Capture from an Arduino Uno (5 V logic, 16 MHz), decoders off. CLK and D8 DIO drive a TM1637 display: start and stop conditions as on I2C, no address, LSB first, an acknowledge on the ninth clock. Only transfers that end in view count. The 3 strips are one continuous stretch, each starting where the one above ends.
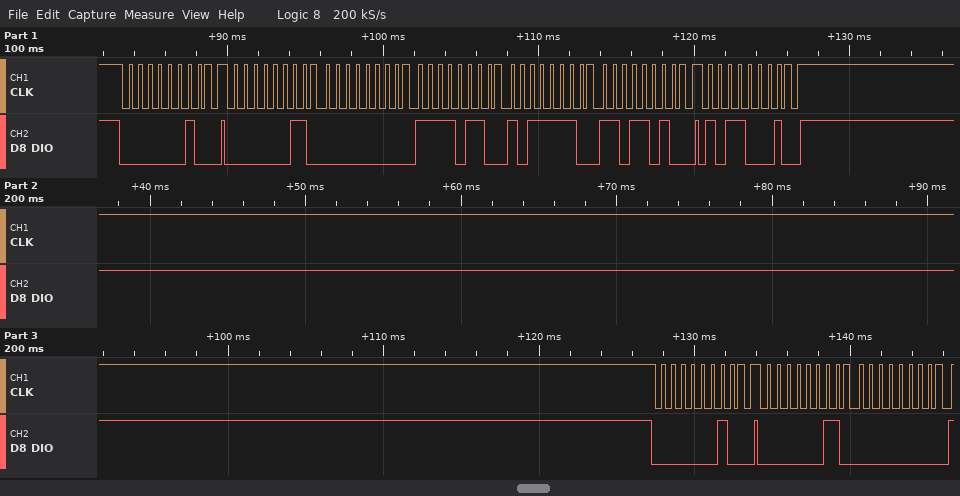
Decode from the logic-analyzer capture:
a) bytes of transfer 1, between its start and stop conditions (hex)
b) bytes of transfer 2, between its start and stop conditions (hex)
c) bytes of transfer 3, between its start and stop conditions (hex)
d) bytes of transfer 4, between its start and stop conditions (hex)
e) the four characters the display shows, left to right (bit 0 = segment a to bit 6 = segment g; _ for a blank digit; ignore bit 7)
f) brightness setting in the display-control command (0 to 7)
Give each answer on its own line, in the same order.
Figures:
40
C0 00 6F 7D 5B
8D
40
_962
5
